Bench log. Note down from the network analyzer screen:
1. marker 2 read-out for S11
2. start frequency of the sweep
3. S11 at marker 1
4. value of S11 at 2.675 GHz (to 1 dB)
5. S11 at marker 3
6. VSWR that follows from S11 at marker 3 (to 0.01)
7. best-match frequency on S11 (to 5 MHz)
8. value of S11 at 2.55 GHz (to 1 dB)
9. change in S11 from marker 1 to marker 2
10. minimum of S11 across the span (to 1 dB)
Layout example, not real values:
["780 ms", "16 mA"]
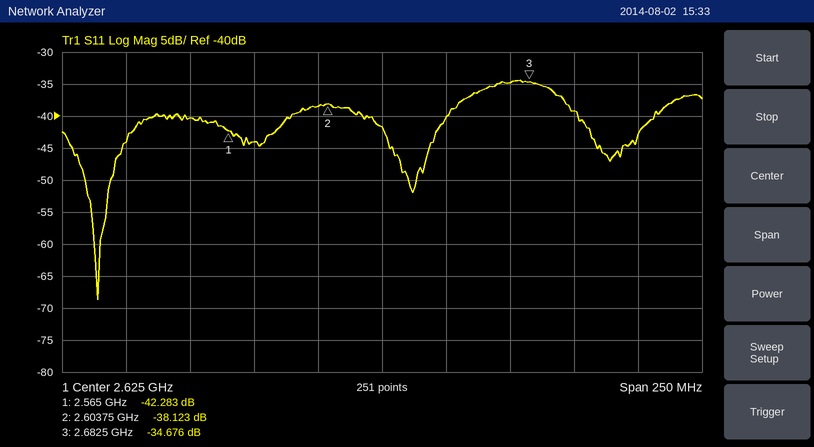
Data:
["-38.123 dB", "2.5 GHz", "-42.283 dB", "-35 dB", "-34.676 dB", "1.04", "2.515 GHz", "-40 dB", "4.160 dB", "-69 dB"]
